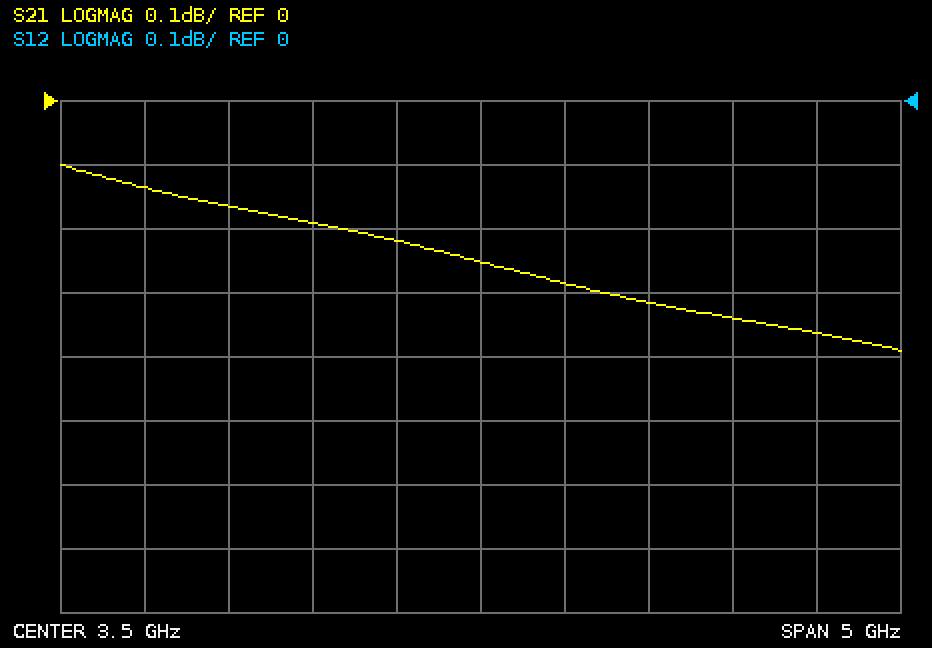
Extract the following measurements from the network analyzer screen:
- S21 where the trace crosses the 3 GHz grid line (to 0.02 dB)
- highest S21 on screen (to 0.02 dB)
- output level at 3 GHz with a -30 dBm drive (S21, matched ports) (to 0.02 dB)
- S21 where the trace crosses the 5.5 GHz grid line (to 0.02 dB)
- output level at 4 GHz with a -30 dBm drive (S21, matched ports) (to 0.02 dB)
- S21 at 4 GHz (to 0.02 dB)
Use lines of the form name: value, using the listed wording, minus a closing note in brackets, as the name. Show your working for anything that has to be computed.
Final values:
S21 where the trace crosses the 3 GHz grid line: -0.22 dB
highest S21 on screen: -0.10 dB
output level at 3 GHz with a -30 dBm drive (S21, matched ports): -30 dBm + (-0.22 dB) = -30.22 dBm
S21 where the trace crosses the 5.5 GHz grid line: -0.36 dB
output level at 4 GHz with a -30 dBm drive (S21, matched ports): -30 dBm + (-0.28 dB) = -30.28 dBm
S21 at 4 GHz: -0.28 dB
